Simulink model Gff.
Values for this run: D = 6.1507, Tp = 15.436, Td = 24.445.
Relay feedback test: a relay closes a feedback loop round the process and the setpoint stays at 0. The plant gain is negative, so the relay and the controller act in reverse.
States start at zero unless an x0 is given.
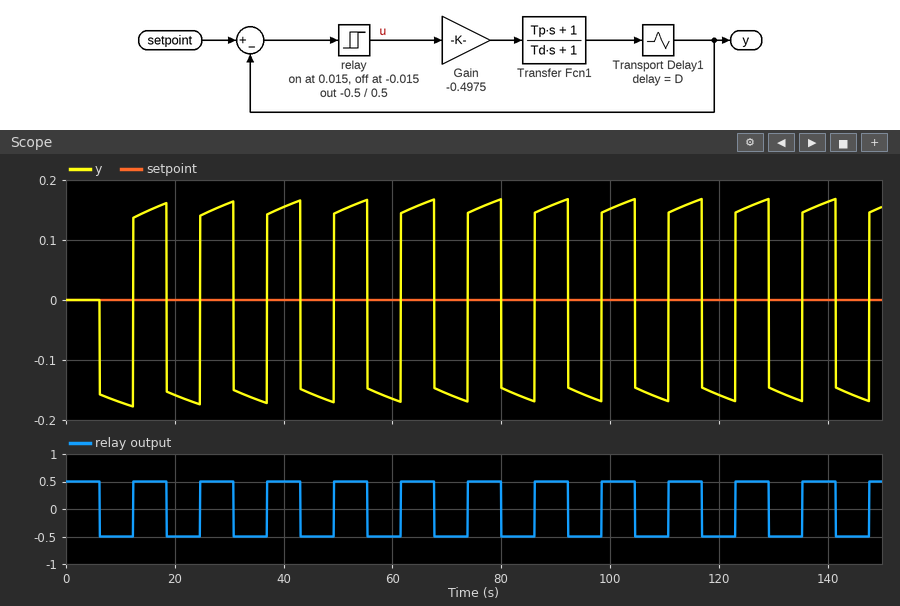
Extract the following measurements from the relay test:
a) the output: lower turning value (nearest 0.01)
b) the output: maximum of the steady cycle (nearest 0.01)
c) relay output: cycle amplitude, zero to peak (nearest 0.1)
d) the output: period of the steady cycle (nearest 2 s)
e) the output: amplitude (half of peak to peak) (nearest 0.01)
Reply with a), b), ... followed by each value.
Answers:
a) -0.17
b) 0.17
c) 0.5
d) 12 s
e) 0.17
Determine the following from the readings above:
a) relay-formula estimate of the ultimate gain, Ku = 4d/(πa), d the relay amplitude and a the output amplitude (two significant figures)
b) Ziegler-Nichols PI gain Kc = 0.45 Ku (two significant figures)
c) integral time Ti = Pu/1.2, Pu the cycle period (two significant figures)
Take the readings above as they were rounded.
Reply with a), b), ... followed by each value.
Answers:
a) 3.7
b) 1.7
c) 10 s
